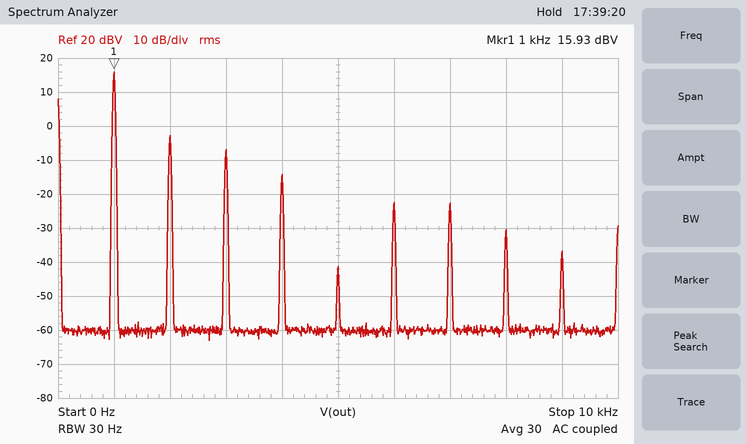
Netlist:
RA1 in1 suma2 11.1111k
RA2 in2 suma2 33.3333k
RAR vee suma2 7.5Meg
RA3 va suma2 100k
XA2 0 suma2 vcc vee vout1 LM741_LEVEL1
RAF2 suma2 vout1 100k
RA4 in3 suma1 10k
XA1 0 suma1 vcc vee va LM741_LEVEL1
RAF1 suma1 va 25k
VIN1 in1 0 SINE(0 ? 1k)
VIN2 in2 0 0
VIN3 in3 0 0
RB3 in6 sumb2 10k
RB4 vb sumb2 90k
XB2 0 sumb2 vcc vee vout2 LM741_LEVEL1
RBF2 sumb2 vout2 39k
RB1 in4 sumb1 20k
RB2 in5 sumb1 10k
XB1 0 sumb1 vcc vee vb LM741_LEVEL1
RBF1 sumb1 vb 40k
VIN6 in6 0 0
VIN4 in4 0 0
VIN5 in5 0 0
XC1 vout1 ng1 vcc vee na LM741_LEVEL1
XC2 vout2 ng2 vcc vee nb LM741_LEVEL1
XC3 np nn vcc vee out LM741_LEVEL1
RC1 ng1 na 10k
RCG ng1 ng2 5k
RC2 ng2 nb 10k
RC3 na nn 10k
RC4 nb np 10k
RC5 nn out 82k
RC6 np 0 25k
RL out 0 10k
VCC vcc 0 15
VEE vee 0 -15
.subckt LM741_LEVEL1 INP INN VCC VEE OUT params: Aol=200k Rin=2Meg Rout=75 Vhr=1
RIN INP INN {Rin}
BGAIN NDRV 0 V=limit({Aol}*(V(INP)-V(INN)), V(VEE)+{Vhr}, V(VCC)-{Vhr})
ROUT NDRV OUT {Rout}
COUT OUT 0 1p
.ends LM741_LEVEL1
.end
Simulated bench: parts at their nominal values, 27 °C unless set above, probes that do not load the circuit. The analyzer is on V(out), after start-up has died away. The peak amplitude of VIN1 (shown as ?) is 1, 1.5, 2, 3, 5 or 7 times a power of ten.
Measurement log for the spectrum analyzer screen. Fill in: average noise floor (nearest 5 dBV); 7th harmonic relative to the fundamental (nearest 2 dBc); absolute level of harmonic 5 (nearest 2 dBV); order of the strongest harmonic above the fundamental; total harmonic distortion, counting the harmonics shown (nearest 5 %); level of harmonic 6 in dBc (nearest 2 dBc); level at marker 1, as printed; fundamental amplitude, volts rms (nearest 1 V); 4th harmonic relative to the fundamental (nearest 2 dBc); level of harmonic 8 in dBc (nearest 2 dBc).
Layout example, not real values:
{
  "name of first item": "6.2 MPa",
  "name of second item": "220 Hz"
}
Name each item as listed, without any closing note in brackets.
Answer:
{
  "average noise floor": "-60 dBV",
  "7th harmonic relative to the fundamental": "-38 dBc",
  "absolute level of harmonic 5": "-42 dBV",
  "order of the strongest harmonic above the fundamental": "2",
  "total harmonic distortion, counting the harmonics shown": "15 %",
  "level of harmonic 6 in dBc": "-38 dBc",
  "level at marker 1, as printed": "15.93 dBV",
  "fundamental amplitude, volts rms": "6 V",
  "4th harmonic relative to the fundamental": "-30 dBc",
  "level of harmonic 8 in dBc": "-46 dBc"
}
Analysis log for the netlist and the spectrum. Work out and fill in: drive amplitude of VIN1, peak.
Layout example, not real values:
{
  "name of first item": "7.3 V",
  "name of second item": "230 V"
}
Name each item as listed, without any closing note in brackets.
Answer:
{
  "drive amplitude of VIN1, peak": "30 mV"
}
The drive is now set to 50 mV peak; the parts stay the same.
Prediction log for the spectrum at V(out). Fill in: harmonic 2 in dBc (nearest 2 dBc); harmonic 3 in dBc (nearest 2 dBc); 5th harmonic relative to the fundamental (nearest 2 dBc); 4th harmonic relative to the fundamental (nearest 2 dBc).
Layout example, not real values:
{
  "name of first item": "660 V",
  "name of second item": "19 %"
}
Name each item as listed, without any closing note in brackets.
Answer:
{
  "harmonic 2 in dBc": "-12 dBc",
  "harmonic 3 in dBc": "-22 dBc",
  "5th harmonic relative to the fundamental": "-30 dBc",
  "4th harmonic relative to the fundamental": "-42 dBc"
}
